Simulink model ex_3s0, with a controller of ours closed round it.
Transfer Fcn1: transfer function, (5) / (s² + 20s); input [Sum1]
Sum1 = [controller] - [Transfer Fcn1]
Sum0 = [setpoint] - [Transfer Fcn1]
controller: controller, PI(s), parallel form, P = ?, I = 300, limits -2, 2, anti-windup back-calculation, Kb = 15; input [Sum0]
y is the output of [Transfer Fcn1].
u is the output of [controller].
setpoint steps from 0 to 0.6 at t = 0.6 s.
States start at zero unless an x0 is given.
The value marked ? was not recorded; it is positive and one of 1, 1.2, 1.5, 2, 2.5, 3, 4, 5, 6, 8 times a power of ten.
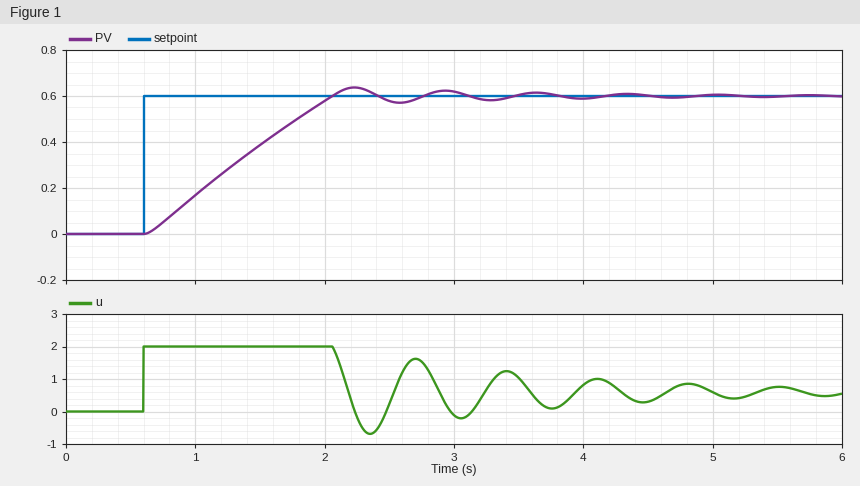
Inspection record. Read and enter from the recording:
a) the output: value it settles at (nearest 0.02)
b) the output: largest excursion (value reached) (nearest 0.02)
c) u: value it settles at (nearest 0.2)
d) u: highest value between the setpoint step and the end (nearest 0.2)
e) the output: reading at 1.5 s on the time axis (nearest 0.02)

0.60
0.64
0.6
2.0
0.38
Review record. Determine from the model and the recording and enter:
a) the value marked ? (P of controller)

20
